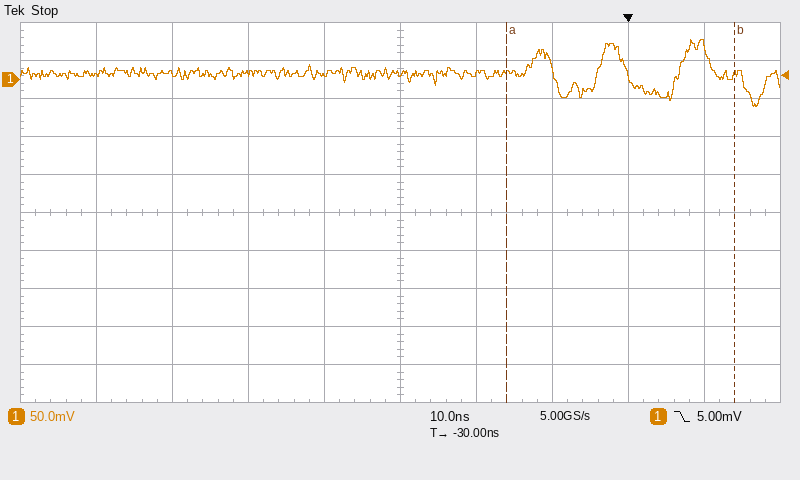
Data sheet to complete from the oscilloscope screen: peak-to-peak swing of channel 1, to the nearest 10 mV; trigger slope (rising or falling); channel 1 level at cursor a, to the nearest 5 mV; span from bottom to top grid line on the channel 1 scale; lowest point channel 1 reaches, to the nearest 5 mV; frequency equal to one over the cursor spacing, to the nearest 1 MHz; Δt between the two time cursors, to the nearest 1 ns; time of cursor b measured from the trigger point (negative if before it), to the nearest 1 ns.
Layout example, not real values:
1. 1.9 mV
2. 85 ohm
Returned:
1. 90 mV
2. falling
3. 10 mV
4. 500 mV
5. -35 mV
6. 33 MHz
7. 30 ns
8. +14 ns
